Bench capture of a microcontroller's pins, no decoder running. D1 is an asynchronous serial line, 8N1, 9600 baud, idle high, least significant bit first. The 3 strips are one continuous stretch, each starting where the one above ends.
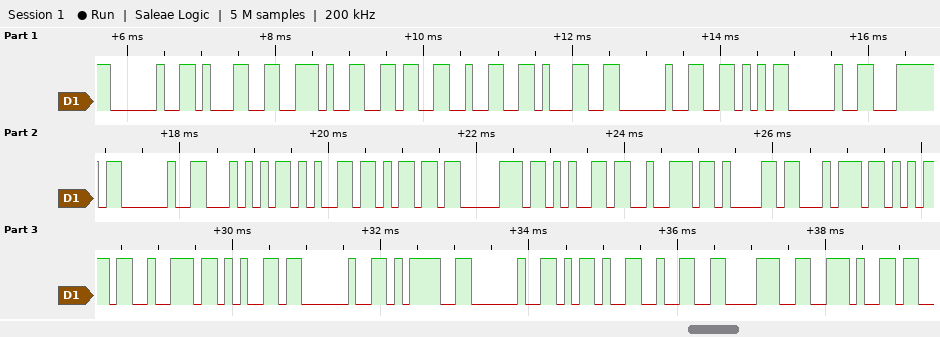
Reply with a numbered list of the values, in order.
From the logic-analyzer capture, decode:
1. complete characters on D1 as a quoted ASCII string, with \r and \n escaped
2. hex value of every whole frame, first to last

1. " 1.621 V | Temperature = -28."
2. 0x20 0x31 0x2E 0x36 0x32 0x31 0x20 0x56 0x20 0x7C 0x20 0x54 0x65 0x6D 0x70 0x65 0x72 0x61 0x74 0x75 0x72 0x65 0x20 0x3D 0x20 0x2D 0x32 0x38 0x2E
